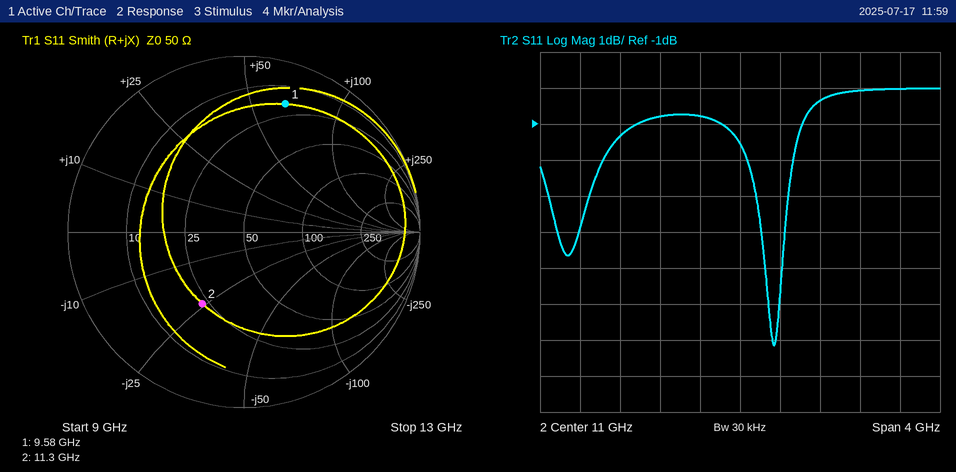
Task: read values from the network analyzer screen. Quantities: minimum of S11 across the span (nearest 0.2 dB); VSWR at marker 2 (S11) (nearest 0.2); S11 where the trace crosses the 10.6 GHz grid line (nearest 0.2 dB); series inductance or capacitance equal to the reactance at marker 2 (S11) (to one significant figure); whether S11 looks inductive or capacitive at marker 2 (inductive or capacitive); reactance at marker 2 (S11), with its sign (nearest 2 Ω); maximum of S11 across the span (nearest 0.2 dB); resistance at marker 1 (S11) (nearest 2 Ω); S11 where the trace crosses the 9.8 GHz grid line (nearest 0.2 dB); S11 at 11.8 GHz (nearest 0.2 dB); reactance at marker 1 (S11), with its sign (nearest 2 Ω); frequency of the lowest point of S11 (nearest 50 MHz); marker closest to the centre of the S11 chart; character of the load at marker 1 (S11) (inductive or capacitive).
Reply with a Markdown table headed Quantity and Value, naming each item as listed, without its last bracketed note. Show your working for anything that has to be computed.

| Quantity | Value |
|---|---|
| minimum of S11 across the span | -7.2 dB |
| VSWR at marker 2 (S11) | 2.8 |
| S11 where the trace crosses the 10.6 GHz grid line | -0.8 dB |
| series inductance or capacitance equal to the reactance at marker 2 (S11) | C = 1/(2π × 11.3 GHz × 24 Ω) ≈ 587 fF, so 600 fF to one significant figure |
| whether S11 looks inductive or capacitive at marker 2 | capacitive |
| reactance at marker 2 (S11), with its sign | -24 Ω |
| maximum of S11 across the span | 0.0 dB |
| resistance at marker 1 (S11) | 18 Ω |
| S11 where the trace crosses the 9.8 GHz grid line | -1.4 dB |
| S11 at 11.8 GHz | -0.4 dB |
| reactance at marker 1 (S11), with its sign | +66 Ω |
| frequency of the lowest point of S11 | 11.35 GHz |
| marker closest to the centre of the S11 chart | marker 2 |
| character of the load at marker 1 (S11) | inductive |
